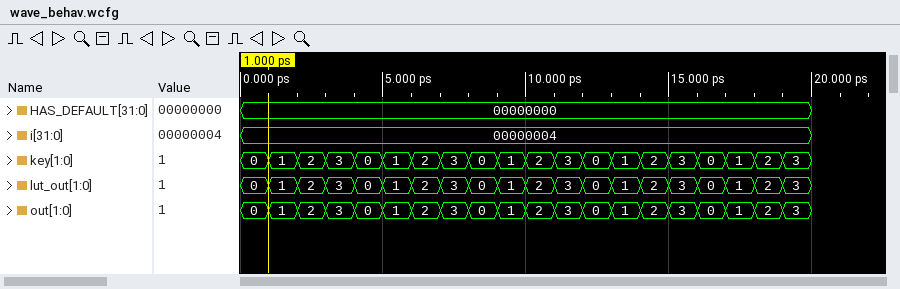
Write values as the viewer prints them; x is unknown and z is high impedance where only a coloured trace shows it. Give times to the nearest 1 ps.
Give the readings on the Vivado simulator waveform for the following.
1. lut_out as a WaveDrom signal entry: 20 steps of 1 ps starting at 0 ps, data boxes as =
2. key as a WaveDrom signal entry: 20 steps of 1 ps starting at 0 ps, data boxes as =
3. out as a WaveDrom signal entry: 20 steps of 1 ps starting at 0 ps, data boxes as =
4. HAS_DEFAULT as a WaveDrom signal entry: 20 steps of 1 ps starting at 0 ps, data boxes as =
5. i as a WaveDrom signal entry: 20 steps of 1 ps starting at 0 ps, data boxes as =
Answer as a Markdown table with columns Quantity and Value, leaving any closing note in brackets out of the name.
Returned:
| Quantity | Value |
|---|---|
| lut_out as a WaveDrom signal entry: 20 steps of 1 ps starting at 0 ps, data boxes as = | {name: 'lut_out', wave: '====================', data: '0 1 2 3 0 1 2 3 0 1 2 3 0 1 2 3 0 1 2 3'} |
| key as a WaveDrom signal entry: 20 steps of 1 ps starting at 0 ps, data boxes as = | {name: 'key', wave: '====================', data: '0 1 2 3 0 1 2 3 0 1 2 3 0 1 2 3 0 1 2 3'} |
| out as a WaveDrom signal entry: 20 steps of 1 ps starting at 0 ps, data boxes as = | {name: 'out', wave: '====================', data: '0 1 2 3 0 1 2 3 0 1 2 3 0 1 2 3 0 1 2 3'} |
| HAS_DEFAULT as a WaveDrom signal entry: 20 steps of 1 ps starting at 0 ps, data boxes as = | {name: 'HAS_DEFAULT', wave: '=...................', data: '00000000'} |
| i as a WaveDrom signal entry: 20 steps of 1 ps starting at 0 ps, data boxes as = | {name: 'i', wave: '=...................', data: '00000004'} |
